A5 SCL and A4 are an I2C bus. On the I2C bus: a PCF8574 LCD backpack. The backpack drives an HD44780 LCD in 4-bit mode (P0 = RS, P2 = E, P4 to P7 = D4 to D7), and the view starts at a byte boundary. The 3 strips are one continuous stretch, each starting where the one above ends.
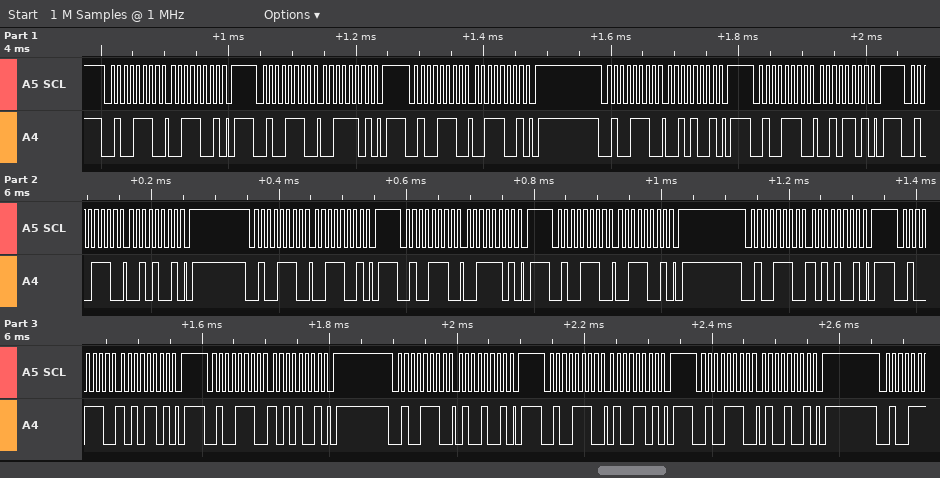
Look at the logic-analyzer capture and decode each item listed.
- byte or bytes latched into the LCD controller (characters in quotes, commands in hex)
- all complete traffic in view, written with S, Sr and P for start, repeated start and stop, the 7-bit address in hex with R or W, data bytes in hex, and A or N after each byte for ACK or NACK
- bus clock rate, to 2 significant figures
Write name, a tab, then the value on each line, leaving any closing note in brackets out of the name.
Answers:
byte or bytes latched into the LCD controller	'2' ':'
all complete traffic in view, written with S, Sr and P for start, repeated start and stop, the 7-bit address in hex with R or W, data bytes in hex, and A or N after each byte for ACK or NACK	S 27W A 39 A P S 27W A 3D A P S 27W A 39 A P S 27W A 29 A P S 27W A 2D A P S 27W A 29 A P S 27W A 39 A P S 27W A 3D A P S 27W A 39 A P S 27W A A9 A P S 27W A AD A P S 27W A A9 A P S 27W A 49 A P S 27W A 4D A P S 27W A 49 A P
bus clock rate, to 2 significant figures	100 kHz
